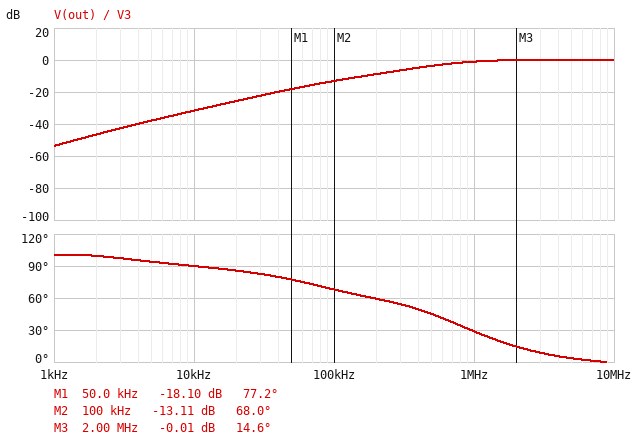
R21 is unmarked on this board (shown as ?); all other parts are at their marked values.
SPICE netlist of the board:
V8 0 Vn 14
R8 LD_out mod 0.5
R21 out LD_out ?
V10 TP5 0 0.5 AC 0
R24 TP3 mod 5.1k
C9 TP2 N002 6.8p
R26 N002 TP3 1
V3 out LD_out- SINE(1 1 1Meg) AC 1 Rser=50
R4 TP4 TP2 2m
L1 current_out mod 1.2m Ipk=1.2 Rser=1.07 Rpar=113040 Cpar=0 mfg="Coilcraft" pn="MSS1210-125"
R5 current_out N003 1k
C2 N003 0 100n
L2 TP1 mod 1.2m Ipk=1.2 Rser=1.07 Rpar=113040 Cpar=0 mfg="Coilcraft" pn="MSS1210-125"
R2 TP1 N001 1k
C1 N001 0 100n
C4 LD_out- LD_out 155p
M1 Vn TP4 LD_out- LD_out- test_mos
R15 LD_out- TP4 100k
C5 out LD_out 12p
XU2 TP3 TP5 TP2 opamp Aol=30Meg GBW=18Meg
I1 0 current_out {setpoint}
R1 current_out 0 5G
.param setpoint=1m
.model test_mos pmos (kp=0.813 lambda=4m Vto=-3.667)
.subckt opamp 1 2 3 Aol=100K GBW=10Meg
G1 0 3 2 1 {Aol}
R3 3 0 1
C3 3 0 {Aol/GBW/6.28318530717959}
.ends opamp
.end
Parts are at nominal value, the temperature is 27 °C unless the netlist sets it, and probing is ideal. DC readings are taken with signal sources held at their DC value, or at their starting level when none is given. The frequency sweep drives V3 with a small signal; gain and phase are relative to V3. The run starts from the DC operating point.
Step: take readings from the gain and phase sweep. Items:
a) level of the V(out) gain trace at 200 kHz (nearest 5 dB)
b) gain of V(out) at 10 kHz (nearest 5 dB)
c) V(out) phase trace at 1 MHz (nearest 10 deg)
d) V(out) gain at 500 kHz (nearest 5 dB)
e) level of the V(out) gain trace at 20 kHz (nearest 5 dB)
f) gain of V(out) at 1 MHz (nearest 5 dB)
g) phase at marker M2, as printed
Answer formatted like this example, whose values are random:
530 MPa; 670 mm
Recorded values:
-10 dB; -30 dB; 30 deg; -5 dB; -25 dB; 0 dB; 68.0 deg
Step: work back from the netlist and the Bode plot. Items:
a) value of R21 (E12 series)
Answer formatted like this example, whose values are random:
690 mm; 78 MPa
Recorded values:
1.5 kΩ
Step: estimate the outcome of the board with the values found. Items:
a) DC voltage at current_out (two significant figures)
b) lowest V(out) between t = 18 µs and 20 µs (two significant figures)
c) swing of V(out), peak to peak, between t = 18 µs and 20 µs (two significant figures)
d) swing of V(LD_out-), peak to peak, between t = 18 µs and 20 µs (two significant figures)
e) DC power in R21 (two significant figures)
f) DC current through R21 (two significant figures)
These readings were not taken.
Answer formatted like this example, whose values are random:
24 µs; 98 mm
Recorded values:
500 mV; -1.9 V; 1.8 V; 970 mV; 1.5 mW; 1.0 mA
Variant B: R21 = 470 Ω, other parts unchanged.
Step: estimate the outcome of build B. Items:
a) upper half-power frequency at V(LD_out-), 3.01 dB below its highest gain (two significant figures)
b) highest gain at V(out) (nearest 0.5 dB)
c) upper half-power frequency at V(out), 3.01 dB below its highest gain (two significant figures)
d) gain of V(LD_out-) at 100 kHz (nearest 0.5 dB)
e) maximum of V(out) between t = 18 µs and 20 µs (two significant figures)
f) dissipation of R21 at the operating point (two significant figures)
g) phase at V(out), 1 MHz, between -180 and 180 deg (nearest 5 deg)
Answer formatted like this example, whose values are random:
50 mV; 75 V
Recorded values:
1.5 MHz; 0.5 dB; 220 MHz; 0 dB; 660 mV; 470 µW; 55 deg
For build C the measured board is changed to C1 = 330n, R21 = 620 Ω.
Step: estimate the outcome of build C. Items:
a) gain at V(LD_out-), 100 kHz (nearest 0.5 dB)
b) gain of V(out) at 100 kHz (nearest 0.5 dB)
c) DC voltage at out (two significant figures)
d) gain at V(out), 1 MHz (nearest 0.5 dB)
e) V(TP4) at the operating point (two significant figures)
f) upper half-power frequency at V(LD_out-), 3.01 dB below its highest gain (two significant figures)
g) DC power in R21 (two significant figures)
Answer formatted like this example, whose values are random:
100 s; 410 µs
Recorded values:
0 dB; -19.0 dB; -120 mV; -3.0 dB; -4.9 V; 1.2 MHz; 620 µW
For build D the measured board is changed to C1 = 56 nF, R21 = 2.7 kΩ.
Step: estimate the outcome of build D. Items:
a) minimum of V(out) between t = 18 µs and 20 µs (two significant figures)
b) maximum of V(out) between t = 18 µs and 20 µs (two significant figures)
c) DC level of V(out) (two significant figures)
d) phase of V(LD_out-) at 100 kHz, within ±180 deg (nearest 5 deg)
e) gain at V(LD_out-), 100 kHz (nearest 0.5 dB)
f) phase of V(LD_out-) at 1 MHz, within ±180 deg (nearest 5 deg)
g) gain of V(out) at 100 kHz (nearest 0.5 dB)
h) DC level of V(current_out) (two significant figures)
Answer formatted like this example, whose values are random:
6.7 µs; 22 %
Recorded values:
-3.1 V; -1.3 V; -2.2 V; 160 deg; -1.0 dB; 110 deg; -9.0 dB; 500 mV
